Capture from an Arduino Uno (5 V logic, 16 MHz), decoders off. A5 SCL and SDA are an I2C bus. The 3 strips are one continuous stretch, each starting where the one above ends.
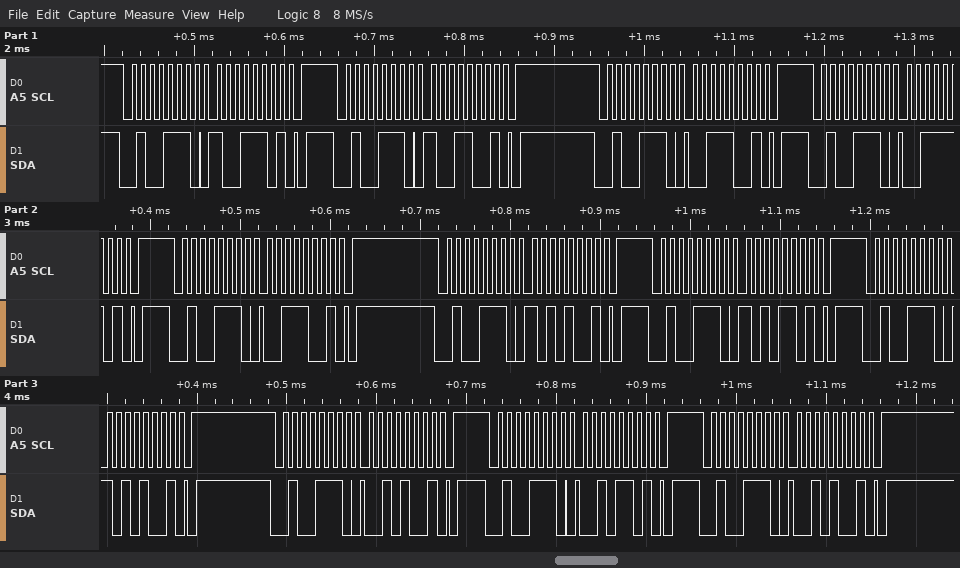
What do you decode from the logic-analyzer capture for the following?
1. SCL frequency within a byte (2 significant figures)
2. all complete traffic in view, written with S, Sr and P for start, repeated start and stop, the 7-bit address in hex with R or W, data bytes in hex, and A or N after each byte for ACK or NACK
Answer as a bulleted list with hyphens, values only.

- 100 kHz
- S 27W A 9D A P S 27W A 99 A P S 27W A 39 A P S 27W A 3D A P S 27W A 39 A P S 27W A A9 A P S 27W A AD A P S 27W A A9 A P S 27W A 29 A P S 27W A 2D A P S 27W A 29 A P
